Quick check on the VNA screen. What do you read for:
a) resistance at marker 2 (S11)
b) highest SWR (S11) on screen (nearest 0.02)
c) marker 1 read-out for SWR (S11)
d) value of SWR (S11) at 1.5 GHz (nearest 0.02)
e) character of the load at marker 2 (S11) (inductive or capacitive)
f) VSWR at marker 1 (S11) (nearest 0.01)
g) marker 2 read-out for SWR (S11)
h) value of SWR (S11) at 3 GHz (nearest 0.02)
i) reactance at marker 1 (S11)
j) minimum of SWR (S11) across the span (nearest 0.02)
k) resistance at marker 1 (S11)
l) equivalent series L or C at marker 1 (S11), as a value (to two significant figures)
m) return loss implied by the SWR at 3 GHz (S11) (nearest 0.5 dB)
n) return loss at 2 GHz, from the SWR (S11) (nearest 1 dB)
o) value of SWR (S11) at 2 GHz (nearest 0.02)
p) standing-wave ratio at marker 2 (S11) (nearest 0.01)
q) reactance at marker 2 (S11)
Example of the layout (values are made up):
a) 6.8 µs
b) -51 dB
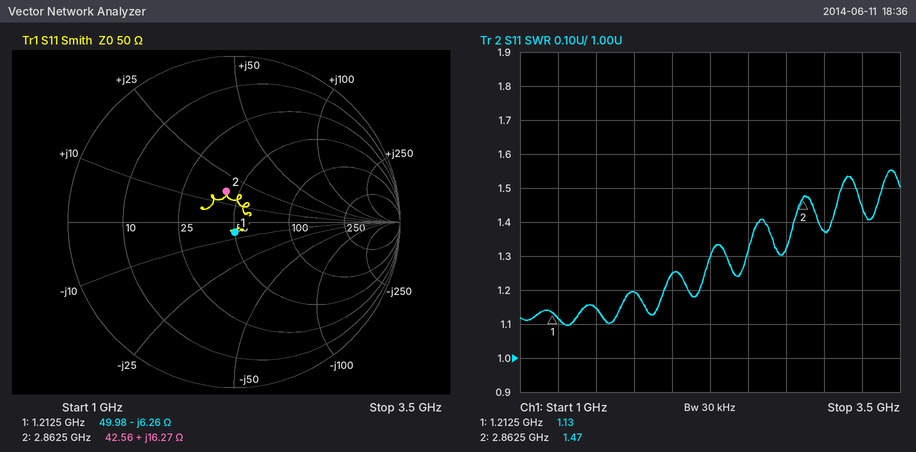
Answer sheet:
a) 42.56 Ω
b) 1.56
c) 1.13
d) 1.14
e) inductive
f) 1.13
g) 1.47
h) 1.38
i) -6.26 Ω
j) 1.10
k) 49.98 Ω
l) 21 pF
m) 16.0 dB
n) 19 dB
o) 1.24
p) 1.47
q) +16.27 Ω
